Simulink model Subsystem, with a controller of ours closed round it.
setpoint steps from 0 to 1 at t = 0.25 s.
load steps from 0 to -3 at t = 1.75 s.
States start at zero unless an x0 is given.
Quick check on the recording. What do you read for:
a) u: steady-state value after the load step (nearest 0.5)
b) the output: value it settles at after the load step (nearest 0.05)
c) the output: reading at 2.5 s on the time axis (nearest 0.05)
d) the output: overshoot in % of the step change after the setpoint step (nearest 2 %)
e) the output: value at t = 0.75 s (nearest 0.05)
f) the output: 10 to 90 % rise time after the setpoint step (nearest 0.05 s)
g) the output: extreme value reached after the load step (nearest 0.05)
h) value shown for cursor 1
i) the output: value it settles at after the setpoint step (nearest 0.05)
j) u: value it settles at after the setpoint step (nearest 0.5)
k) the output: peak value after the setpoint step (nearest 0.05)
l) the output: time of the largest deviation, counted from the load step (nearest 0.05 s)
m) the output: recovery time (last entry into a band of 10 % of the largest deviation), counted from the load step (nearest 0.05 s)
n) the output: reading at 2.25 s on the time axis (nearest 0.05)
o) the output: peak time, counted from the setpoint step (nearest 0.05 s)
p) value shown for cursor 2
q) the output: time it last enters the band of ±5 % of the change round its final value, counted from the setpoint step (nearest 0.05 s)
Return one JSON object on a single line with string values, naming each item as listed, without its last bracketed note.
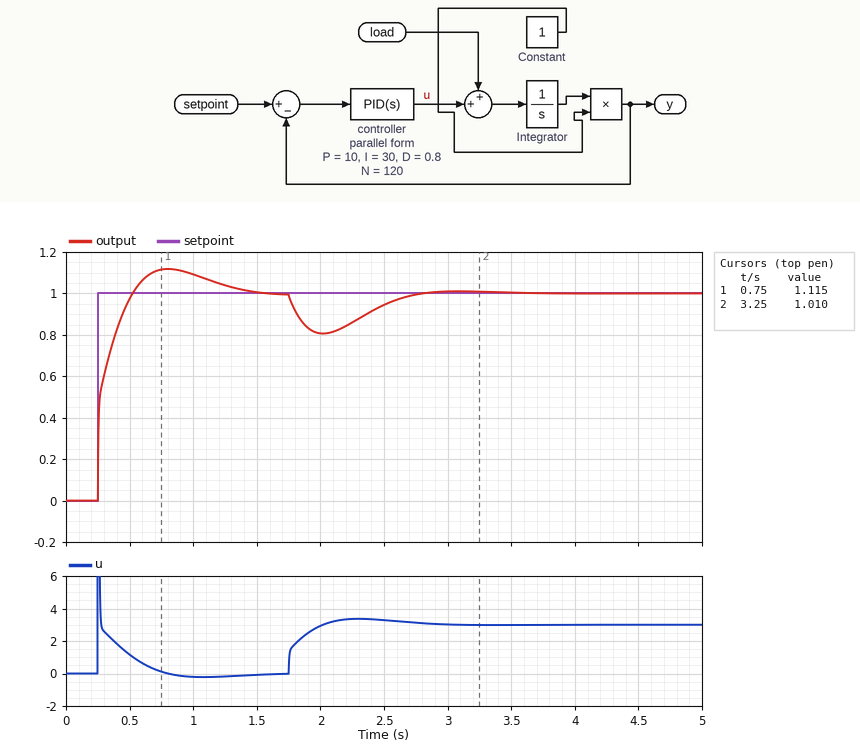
{"u: steady-state value after the load step": "3.0", "the output: value it settles at after the load step": "1.00", "the output: reading at 2.5 s on the time axis": "0.95", "the output: overshoot in % of the step change after the setpoint step": "12 %", "the output: value at t = 0.75 s": "1.10", "the output: 10 to 90 % rise time after the setpoint step": "0.20 s", "the output: extreme value reached after the load step": "0.80", "value shown for cursor 1": "1.115", "the output: value it settles at after the setpoint step": "1.00", "u: value it settles at after the setpoint step": "0.0", "the output: peak value after the setpoint step": "1.10", "the output: time of the largest deviation, counted from the load step": "0.25 s", "the output: recovery time (last entry into a band of 10 % of the largest deviation), counted from the load step": "0.90 s", "the output: reading at 2.25 s on the time axis": "0.85", "the output: peak time, counted from the setpoint step": "0.55 s", "value shown for cursor 2": "1.010", "the output: time it last enters the band of ±5 % of the change round its final value, counted from the setpoint step": "0.95 s"}
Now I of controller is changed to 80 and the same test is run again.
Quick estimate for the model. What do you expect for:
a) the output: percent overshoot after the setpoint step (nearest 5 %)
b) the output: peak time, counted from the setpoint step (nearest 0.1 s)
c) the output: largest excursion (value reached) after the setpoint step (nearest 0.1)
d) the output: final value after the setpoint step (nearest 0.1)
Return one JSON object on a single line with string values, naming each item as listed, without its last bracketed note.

{"the output: percent overshoot after the setpoint step": "20 %", "the output: peak time, counted from the setpoint step": "0.4 s", "the output: largest excursion (value reached) after the setpoint step": "1.2", "the output: final value after the setpoint step": "1.0"}
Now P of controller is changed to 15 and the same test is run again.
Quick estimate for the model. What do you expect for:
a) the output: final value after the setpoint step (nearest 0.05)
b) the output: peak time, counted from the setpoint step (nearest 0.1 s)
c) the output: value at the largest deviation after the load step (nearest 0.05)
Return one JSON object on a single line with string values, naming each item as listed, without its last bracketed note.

{"the output: final value after the setpoint step": "1.00", "the output: peak time, counted from the setpoint step": "0.5 s", "the output: value at the largest deviation after the load step": "0.85"}
